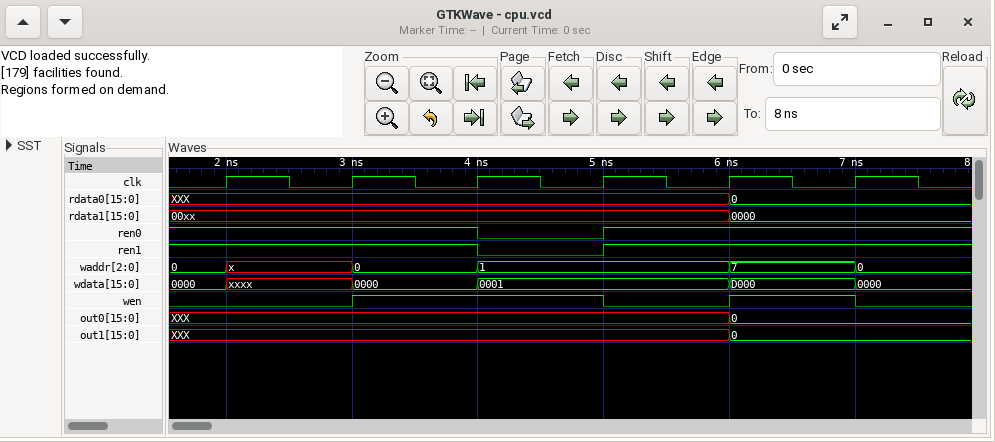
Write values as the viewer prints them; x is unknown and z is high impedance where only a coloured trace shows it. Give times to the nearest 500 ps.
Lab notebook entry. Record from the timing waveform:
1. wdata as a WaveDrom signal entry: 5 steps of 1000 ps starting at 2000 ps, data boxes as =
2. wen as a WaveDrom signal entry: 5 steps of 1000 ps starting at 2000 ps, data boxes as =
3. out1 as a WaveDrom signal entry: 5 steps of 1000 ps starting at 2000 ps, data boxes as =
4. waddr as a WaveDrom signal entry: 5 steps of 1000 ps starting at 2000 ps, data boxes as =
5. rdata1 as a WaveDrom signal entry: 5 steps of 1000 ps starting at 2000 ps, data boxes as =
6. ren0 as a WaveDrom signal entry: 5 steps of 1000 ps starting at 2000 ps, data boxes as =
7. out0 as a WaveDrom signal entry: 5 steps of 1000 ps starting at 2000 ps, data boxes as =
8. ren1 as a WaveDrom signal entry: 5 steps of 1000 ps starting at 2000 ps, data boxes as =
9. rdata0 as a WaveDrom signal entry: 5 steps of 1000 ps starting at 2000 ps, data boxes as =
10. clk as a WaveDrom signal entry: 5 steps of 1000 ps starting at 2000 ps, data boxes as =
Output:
{name: 'wdata', wave: 'x==.=', data: '0000 0001 D000'}
{name: 'wen', wave: '01.01'}
{name: 'out1', wave: '=...=', data: 'XXX 0'}
{name: 'waddr', wave: 'x==.=', data: '0 1 7'}
{name: 'rdata1', wave: '=...=', data: '00xx 0000'}
{name: 'ren0', wave: '1.01.'}
{name: 'out0', wave: '=...=', data: 'XXX 0'}
{name: 'ren1', wave: '1.01.'}
{name: 'rdata0', wave: '=...=', data: 'XXX 0'}
{name: 'clk', wave: 'p....'}
